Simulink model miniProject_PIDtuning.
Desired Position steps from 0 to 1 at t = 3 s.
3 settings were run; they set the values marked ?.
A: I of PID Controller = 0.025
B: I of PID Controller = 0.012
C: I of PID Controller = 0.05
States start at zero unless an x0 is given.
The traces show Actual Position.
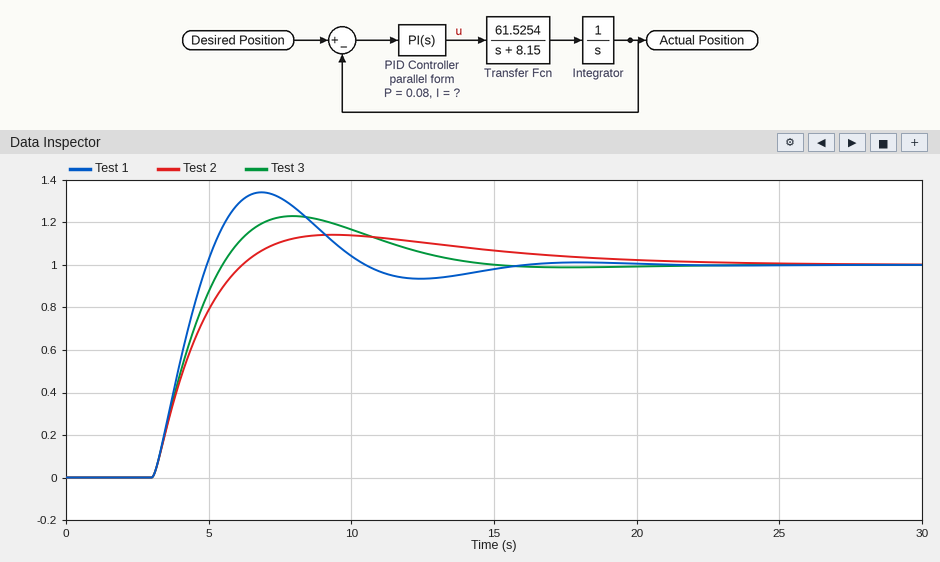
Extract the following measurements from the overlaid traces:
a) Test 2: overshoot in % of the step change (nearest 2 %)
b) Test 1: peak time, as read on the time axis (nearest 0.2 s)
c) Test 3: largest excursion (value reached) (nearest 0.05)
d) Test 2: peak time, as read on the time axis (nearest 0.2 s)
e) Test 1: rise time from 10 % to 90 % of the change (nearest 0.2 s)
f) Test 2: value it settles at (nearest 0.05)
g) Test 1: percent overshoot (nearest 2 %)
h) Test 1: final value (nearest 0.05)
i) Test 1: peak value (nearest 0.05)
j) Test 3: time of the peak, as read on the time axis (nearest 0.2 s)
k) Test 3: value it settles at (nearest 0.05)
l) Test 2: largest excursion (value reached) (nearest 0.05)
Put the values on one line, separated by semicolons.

14 %; 6.8 s; 1.25; 9.4 s; 1.4 s; 1.00; 34 %; 1.00; 1.35; 8.0 s; 1.00; 1.15
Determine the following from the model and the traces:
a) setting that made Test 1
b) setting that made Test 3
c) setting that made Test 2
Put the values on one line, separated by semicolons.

C; A; B
